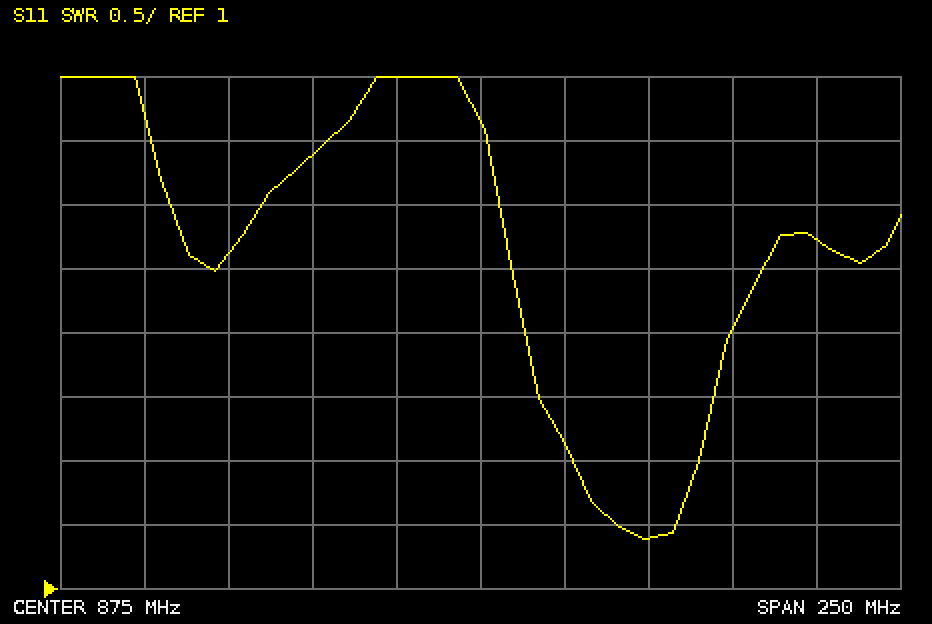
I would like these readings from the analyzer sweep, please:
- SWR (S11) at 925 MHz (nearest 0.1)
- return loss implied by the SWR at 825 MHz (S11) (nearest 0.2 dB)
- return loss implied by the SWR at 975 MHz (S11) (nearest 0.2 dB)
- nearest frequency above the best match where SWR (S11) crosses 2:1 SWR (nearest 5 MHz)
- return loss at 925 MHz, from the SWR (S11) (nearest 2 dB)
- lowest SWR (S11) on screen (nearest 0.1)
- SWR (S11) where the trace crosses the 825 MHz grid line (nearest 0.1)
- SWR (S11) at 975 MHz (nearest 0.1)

1.4
4.0 dB
4.8 dB
940 MHz
16 dB
1.4
4.4
3.7
